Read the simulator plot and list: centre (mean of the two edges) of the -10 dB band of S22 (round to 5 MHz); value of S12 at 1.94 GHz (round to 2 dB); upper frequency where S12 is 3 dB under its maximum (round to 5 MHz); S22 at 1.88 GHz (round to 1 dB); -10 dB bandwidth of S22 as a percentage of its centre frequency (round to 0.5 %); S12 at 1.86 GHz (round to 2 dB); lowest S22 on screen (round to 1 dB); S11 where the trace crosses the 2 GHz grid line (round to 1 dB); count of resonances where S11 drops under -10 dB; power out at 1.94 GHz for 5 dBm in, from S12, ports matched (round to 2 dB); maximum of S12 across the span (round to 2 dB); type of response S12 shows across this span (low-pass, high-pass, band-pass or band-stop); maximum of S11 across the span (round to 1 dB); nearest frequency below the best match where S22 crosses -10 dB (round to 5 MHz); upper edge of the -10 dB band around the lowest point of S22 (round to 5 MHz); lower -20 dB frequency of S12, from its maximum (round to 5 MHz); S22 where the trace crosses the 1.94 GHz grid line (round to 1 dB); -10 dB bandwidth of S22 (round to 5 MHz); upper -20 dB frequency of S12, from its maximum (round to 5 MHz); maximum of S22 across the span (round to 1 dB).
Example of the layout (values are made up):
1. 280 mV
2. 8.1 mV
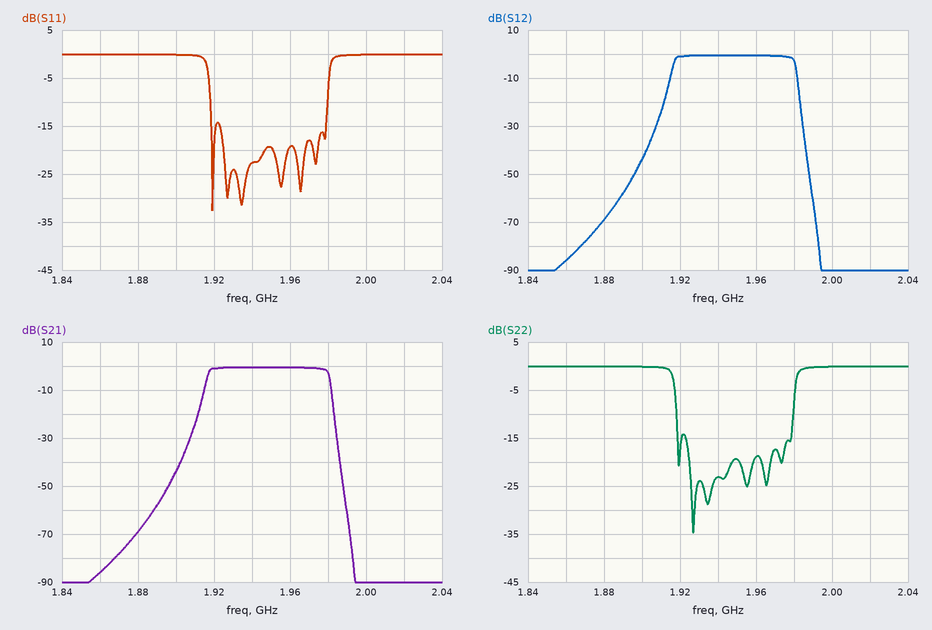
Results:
1. 1.950 GHz
2. 0 dB
3. 1.980 GHz
4. 0 dB
5. 3.0 %
6. -86 dB
7. -35 dB
8. 0 dB
9. 6
10. 4 dBm
11. 0 dB
12. band-pass
13. 0 dB
14. 1.920 GHz
15. 1.980 GHz
16. 1.910 GHz
17. -23 dB
18. 60 MHz
19. 1.985 GHz
20. 0 dB
